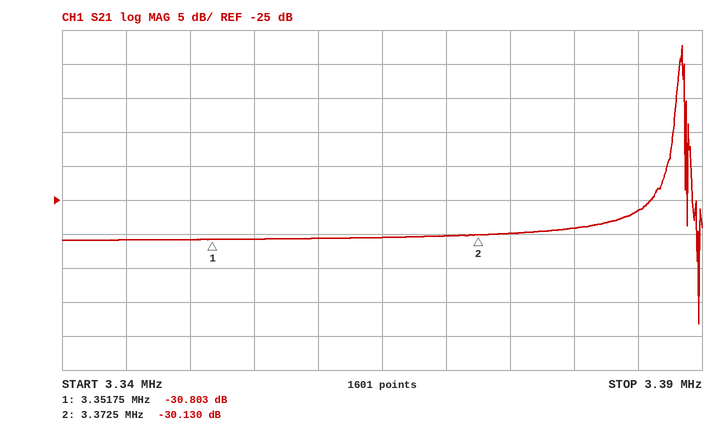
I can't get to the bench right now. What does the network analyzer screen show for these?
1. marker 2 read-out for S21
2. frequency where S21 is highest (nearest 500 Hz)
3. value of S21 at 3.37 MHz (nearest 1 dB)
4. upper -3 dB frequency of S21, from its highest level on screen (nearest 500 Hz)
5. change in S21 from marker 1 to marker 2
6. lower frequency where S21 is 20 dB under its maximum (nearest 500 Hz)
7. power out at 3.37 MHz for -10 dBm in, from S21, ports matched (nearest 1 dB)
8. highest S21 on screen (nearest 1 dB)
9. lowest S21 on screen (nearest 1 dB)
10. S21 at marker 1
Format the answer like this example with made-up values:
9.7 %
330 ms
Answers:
-30.130 dB
3.3885 MHz
-30 dB
3.3885 MHz
0.673 dB
3.3870 MHz
-40 dBm
-2 dB
-43 dB
-30.803 dB
